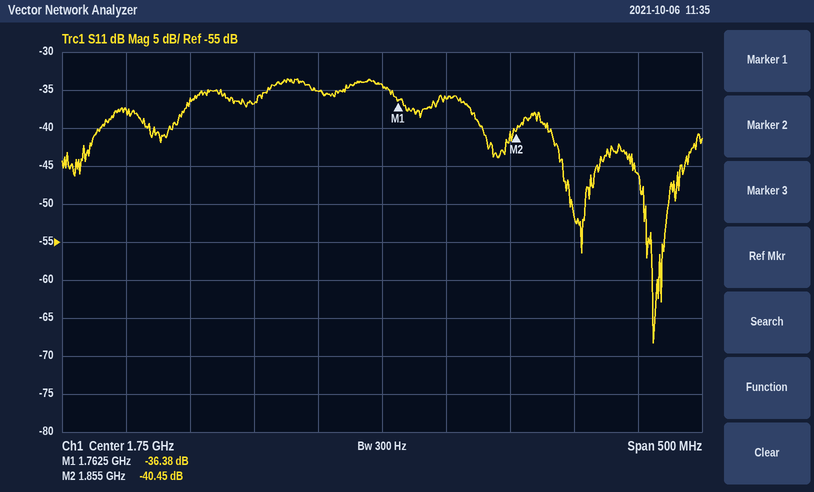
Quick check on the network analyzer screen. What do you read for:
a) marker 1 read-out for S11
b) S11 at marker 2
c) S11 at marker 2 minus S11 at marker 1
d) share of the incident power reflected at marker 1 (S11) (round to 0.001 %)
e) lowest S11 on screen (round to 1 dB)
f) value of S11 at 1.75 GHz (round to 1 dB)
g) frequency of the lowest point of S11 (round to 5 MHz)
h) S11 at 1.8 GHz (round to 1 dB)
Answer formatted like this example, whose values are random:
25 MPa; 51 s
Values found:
-36.38 dB; -40.45 dB; -4.07 dB; 0.023 %; -68 dB; -34 dB; 1.960 GHz; -36 dB
